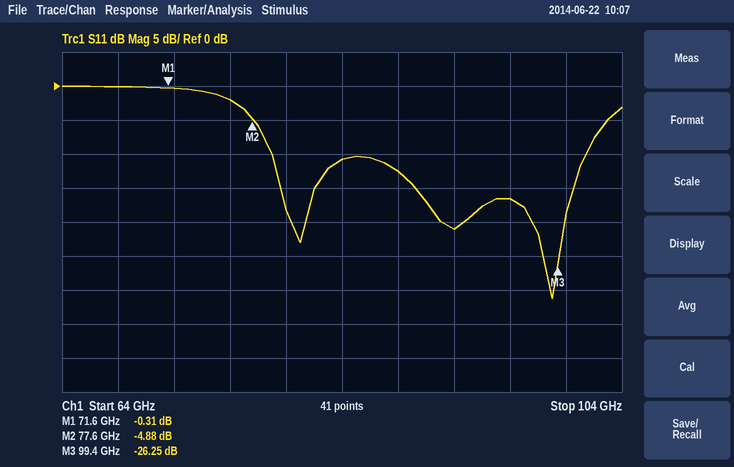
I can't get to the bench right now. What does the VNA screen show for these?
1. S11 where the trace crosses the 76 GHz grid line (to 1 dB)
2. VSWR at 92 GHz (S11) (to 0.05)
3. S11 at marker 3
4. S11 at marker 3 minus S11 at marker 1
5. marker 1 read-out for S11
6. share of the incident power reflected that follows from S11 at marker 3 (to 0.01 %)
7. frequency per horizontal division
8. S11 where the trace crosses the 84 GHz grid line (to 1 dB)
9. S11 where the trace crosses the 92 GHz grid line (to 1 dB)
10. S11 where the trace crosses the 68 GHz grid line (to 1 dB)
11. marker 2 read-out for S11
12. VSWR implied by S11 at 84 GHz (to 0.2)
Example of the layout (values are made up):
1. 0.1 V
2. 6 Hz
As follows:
1. -2 dB
2. 1.20
3. -26.25 dB
4. -25.94 dB
5. -0.31 dB
6. 0.24 %
7. 4 GHz
8. -11 dB
9. -21 dB
10. 0 dB
11. -4.88 dB
12. 1.8
